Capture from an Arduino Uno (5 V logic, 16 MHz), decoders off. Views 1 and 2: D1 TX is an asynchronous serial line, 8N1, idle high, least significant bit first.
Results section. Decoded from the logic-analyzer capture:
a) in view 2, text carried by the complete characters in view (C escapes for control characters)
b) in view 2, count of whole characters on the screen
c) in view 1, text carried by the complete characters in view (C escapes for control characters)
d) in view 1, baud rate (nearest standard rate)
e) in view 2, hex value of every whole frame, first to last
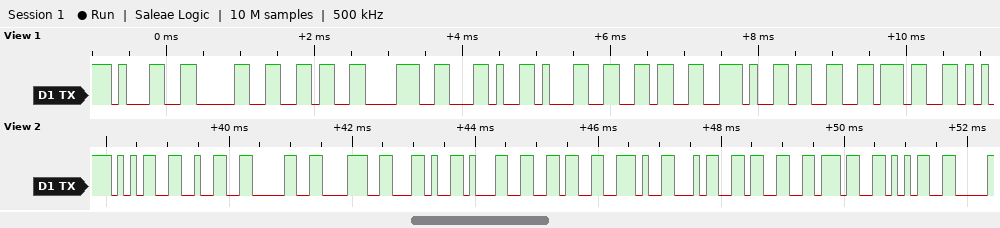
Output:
"5208,16.4375"
12
"1068,16.37"
9600 baud
0x35 0x32 0x30 0x38 0x2C 0x31 0x36 0x2E 0x34 0x33 0x37 0x35
